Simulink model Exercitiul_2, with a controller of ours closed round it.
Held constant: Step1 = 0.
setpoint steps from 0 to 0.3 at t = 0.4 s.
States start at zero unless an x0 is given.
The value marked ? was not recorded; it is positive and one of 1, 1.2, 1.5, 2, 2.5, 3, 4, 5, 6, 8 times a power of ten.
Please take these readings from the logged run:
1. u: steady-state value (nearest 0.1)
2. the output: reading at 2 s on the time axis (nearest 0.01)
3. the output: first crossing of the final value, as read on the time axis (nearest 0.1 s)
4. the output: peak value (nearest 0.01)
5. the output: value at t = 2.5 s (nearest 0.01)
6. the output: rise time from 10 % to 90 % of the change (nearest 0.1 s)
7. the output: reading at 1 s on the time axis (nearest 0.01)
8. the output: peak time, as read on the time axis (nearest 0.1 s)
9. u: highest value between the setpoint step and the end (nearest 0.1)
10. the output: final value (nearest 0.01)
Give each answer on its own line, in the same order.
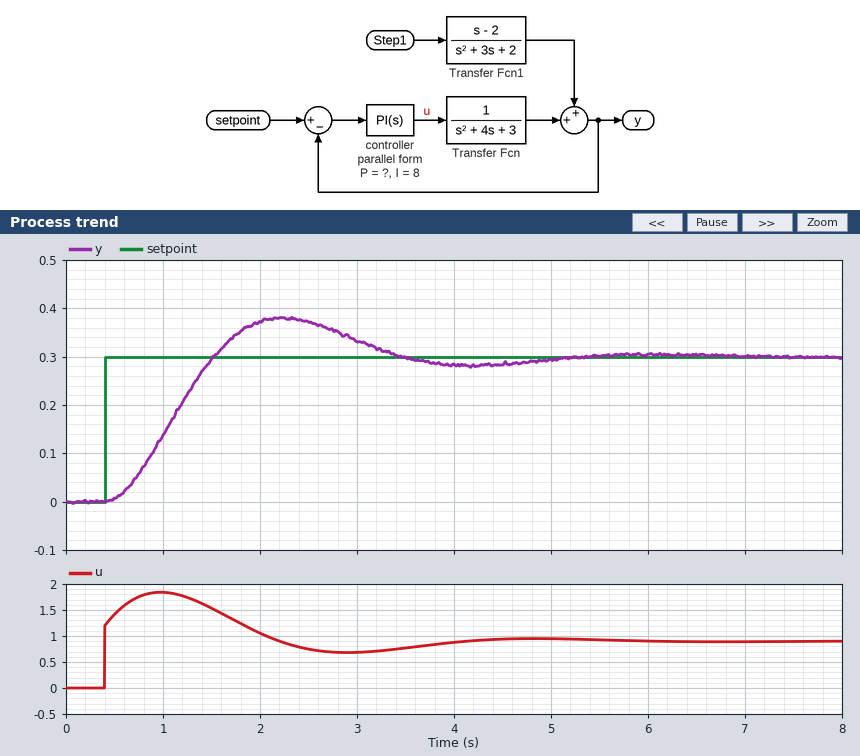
0.9
0.37
1.5 s
0.38
0.37
0.8 s
0.14
2.2 s
1.8
0.30
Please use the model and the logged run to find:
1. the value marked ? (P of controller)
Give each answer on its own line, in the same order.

4
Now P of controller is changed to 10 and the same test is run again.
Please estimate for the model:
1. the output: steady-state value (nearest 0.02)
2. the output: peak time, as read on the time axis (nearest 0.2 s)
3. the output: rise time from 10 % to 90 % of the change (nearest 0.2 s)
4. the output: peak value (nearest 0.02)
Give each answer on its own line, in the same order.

0.30
1.6 s
0.6 s
0.34
